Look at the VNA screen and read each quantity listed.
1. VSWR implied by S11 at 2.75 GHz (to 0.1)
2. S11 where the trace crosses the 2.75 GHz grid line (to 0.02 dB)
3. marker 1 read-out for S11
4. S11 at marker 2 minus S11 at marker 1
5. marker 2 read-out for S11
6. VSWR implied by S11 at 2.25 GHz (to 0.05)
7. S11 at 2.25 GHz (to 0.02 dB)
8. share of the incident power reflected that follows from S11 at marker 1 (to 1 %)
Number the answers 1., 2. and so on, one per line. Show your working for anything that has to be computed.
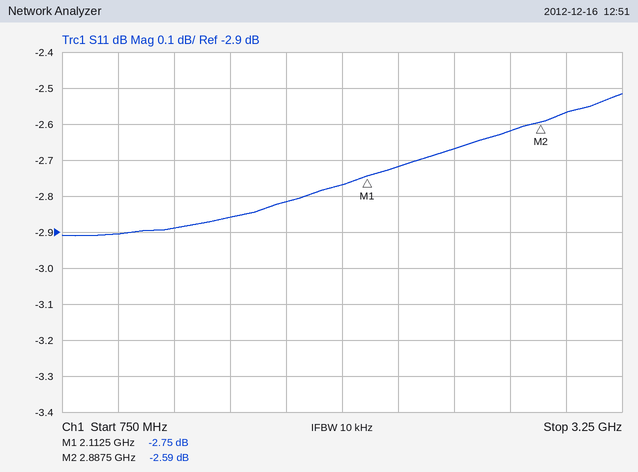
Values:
1. |Γ| = 10^(-2.62/20) = 0.7396; VSWR = (1 + 0.7396)/(1 − 0.7396) ≈ 6.7
2. -2.62 dB
3. -2.75 dB
4. -2.59 − (-2.75) = 0.16 dB
5. -2.59 dB
6. |Γ| = 10^(-2.72/20) = 0.7311; VSWR = (1 + 0.7311)/(1 − 0.7311) ≈ 6.44, so 6.45 to the nearest 0.05
7. -2.72 dB
8. 10^(-2.75/10) ≈ 53 %
